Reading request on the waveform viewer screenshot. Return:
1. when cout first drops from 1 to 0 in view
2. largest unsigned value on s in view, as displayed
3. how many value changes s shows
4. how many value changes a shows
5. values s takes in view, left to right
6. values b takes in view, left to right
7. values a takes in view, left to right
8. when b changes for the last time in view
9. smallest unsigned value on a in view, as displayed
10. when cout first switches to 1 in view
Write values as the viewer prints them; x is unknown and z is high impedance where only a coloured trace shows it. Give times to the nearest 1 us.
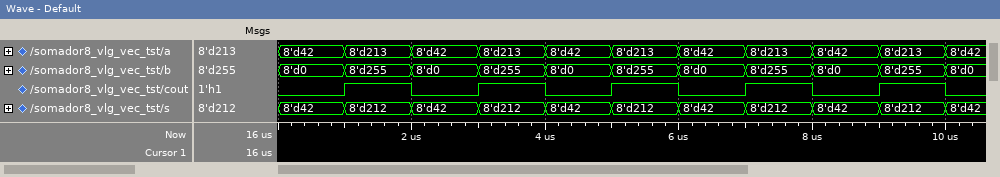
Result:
2 us
8'd212
10
10
8'd42, 8'd212, 8'd42, 8'd212, 8'd42, 8'd212, 8'd42, 8'd212, 8'd42, 8'd212, 8'd42
8'd0, 8'd255, 8'd0, 8'd255, 8'd0, 8'd255, 8'd0, 8'd255, 8'd0, 8'd255, 8'd0
8'd42, 8'd213, 8'd42, 8'd213, 8'd42, 8'd213, 8'd42, 8'd213, 8'd42, 8'd213, 8'd42
10 us
8'd42
1 us
